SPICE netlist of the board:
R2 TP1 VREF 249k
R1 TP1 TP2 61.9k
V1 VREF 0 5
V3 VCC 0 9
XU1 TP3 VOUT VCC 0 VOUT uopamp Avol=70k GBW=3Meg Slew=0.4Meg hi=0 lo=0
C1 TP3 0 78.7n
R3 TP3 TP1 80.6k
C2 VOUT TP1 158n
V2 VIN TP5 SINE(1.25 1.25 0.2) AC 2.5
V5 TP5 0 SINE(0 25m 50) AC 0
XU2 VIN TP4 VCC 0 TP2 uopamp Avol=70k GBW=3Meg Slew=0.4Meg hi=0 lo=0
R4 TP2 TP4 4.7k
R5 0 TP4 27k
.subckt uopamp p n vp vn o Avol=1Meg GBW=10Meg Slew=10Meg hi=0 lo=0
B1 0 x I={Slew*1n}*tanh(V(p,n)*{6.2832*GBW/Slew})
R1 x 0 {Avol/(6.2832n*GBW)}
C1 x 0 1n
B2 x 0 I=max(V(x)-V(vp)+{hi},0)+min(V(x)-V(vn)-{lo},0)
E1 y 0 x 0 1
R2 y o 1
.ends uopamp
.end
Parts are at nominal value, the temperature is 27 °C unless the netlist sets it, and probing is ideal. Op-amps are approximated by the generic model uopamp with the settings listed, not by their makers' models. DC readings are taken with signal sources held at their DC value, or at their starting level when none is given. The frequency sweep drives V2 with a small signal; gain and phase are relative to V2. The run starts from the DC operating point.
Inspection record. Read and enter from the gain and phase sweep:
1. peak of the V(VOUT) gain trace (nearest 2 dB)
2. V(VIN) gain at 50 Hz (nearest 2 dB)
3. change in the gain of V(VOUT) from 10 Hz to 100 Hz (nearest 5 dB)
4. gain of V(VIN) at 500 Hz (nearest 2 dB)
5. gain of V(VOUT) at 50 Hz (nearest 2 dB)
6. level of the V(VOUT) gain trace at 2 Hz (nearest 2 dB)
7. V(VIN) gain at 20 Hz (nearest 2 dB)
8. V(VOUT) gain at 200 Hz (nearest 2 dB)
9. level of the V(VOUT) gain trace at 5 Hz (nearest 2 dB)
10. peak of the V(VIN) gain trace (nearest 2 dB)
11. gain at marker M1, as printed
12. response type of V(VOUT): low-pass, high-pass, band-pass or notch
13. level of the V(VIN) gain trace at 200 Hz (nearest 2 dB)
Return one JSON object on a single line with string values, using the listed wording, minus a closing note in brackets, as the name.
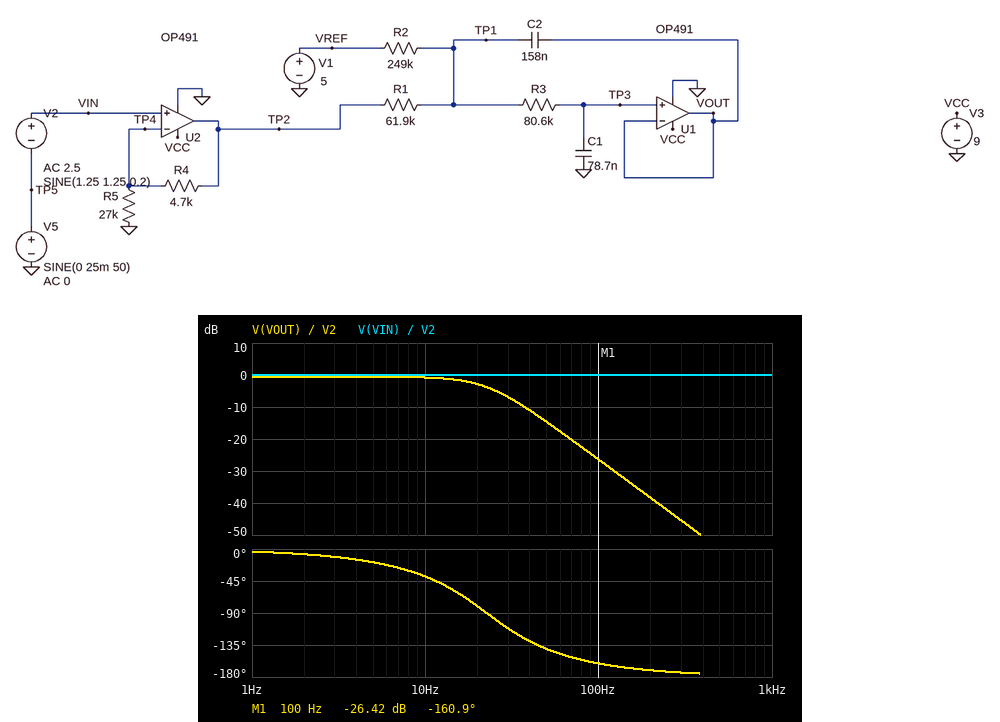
{"peak of the V(VOUT) gain trace": "0 dB", "V(VIN) gain at 50 Hz": "0 dB", "change in the gain of V(VOUT) from 10 Hz to 100 Hz": "-25 dB", "gain of V(VIN) at 500 Hz": "0 dB", "gain of V(VOUT) at 50 Hz": "-14 dB", "level of the V(VOUT) gain trace at 2 Hz": "0 dB", "V(VIN) gain at 20 Hz": "0 dB", "V(VOUT) gain at 200 Hz": "-38 dB", "level of the V(VOUT) gain trace at 5 Hz": "0 dB", "peak of the V(VIN) gain trace": "0 dB", "gain at marker M1, as printed": "-26.42 dB", "response type of V(VOUT): low-pass, high-pass, band-pass or notch": "low-pass", "level of the V(VIN) gain trace at 200 Hz": "0 dB"}
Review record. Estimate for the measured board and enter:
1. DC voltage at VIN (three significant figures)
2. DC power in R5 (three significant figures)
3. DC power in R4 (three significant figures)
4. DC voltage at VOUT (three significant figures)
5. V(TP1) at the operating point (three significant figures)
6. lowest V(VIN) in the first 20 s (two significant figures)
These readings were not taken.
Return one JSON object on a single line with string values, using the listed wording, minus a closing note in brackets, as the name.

{"DC voltage at VIN": "1.25 V", "DC power in R5": "57.9 µW", "DC power in R4": "10.1 µW", "DC voltage at VOUT": "2.17 V", "V(TP1) at the operating point": "2.17 V", "lowest V(VIN) in the first 20 s": "-25 mV"}
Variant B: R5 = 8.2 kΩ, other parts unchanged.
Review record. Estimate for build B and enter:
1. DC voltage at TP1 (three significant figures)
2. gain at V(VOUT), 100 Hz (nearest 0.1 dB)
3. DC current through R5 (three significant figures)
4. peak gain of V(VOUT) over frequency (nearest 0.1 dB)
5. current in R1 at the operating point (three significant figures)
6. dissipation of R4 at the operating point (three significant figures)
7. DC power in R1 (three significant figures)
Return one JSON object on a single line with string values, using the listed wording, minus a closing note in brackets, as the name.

{"DC voltage at TP1": "2.57 V", "gain at V(VOUT), 100 Hz": "-23.9 dB", "DC current through R5": "152 µA", "peak gain of V(VOUT) over frequency": "2.0 dB", "current in R1 at the operating point": "9.76 µA", "dissipation of R4 at the operating point": "109 µW", "DC power in R1": "5.89 µW"}
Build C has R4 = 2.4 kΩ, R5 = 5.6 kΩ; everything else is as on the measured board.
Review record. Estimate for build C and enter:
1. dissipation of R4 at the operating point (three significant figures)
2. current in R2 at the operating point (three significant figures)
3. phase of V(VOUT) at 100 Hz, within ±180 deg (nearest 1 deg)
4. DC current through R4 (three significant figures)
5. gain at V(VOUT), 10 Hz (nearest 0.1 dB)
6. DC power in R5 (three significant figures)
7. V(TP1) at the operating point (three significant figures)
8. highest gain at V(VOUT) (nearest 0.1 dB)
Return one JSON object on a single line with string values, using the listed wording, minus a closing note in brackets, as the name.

{"dissipation of R4 at the operating point": "120 µW", "current in R2 at the operating point": "10.3 µA", "phase of V(VOUT) at 100 Hz, within ±180 deg": "-161 deg", "DC current through R4": "223 µA", "gain at V(VOUT), 10 Hz": "0.9 dB", "DC power in R5": "279 µW", "V(TP1) at the operating point": "2.43 V", "highest gain at V(VOUT)": "1.2 dB"}
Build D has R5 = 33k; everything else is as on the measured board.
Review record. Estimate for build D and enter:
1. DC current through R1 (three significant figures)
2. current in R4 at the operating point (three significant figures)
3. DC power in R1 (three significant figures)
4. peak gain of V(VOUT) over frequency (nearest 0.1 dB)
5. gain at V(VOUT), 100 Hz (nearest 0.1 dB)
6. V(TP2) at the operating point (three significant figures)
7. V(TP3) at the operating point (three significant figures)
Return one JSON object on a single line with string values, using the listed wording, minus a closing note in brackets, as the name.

{"DC current through R1": "11.5 µA", "current in R4 at the operating point": "37.9 µA", "DC power in R1": "8.17 µW", "peak gain of V(VOUT) over frequency": "-0.8 dB", "gain at V(VOUT), 100 Hz": "-26.7 dB", "V(TP2) at the operating point": "1.43 V", "V(TP3) at the operating point": "2.14 V"}
